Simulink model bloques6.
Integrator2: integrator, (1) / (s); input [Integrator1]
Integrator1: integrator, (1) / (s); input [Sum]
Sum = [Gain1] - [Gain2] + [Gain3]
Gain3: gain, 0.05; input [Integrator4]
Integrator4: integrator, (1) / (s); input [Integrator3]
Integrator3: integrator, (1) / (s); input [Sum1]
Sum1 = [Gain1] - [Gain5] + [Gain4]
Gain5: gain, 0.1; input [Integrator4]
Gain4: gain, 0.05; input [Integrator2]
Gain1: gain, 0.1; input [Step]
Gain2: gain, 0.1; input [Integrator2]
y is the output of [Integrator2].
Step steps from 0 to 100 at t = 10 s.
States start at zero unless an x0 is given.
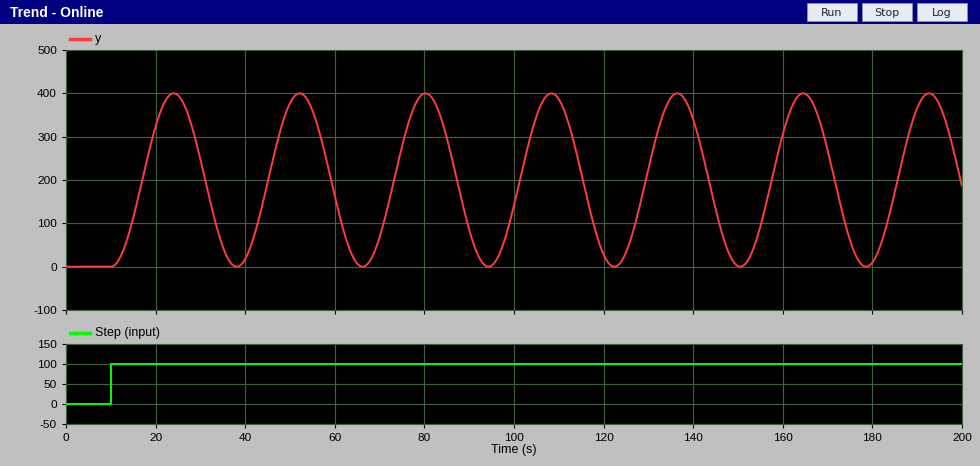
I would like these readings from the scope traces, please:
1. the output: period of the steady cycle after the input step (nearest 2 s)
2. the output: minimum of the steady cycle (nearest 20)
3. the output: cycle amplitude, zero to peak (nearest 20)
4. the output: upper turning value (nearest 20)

28 s
0
200
400
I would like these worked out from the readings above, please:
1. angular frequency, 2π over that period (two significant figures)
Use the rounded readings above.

0.22 rad/s
